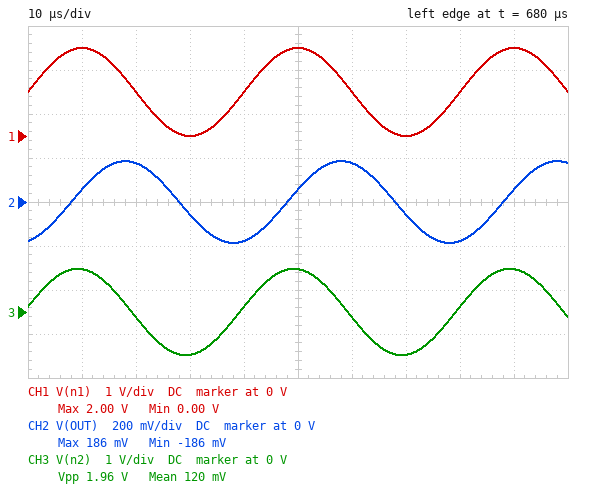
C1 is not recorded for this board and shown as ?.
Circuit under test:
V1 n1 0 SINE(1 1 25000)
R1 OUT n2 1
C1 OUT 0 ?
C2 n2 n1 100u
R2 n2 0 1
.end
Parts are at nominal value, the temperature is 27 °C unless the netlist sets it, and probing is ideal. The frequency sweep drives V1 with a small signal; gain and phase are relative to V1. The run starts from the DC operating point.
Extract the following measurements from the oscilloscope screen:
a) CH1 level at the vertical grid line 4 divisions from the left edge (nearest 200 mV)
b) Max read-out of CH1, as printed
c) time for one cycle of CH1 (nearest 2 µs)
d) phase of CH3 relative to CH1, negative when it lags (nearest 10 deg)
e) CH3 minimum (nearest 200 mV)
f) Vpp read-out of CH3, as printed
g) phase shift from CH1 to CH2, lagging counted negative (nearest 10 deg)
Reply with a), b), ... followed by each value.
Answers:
a) 1.0 V
b) 2.00 V
c) 40 µs
d) 10 deg
e) -1.0 V
f) 1.96 V
g) -70 deg
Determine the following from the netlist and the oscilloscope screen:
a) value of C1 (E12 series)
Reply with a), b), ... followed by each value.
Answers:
a) 33 µF
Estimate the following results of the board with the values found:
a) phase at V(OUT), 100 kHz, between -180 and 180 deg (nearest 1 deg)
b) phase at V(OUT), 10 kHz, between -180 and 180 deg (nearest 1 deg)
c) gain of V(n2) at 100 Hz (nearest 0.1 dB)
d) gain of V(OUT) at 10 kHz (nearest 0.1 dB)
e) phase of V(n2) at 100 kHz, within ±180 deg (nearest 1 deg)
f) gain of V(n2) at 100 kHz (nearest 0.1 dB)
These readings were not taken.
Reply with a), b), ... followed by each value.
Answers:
a) -85 deg
b) -49 deg
c) -24.1 dB
d) -8.1 dB
e) 2 deg
f) 0 dB
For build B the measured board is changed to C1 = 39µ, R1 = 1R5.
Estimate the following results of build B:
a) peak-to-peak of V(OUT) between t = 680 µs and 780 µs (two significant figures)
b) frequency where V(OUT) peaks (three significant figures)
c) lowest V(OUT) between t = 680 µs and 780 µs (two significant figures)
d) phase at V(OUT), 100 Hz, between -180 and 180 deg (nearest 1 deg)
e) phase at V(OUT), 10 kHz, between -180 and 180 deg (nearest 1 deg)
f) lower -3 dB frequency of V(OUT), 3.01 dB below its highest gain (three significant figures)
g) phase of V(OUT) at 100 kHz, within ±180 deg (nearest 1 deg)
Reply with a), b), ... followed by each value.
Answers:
a) 210 mV
b) 2.08 kHz
c) -110 mV
d) 83 deg
e) -61 deg
f) 712 Hz
g) -87 deg
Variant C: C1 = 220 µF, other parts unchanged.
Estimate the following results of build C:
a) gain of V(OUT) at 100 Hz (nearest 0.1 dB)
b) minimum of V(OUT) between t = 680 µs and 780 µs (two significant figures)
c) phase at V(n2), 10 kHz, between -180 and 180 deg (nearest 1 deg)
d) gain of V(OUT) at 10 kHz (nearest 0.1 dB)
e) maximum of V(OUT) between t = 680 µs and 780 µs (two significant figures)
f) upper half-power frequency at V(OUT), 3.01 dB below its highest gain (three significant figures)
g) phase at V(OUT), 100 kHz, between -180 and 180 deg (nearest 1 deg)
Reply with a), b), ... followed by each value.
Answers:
a) -24.4 dB
b) -29 mV
c) 17 deg
d) -23.3 dB
e) 28 mV
f) 4.18 kHz
g) -88 deg
